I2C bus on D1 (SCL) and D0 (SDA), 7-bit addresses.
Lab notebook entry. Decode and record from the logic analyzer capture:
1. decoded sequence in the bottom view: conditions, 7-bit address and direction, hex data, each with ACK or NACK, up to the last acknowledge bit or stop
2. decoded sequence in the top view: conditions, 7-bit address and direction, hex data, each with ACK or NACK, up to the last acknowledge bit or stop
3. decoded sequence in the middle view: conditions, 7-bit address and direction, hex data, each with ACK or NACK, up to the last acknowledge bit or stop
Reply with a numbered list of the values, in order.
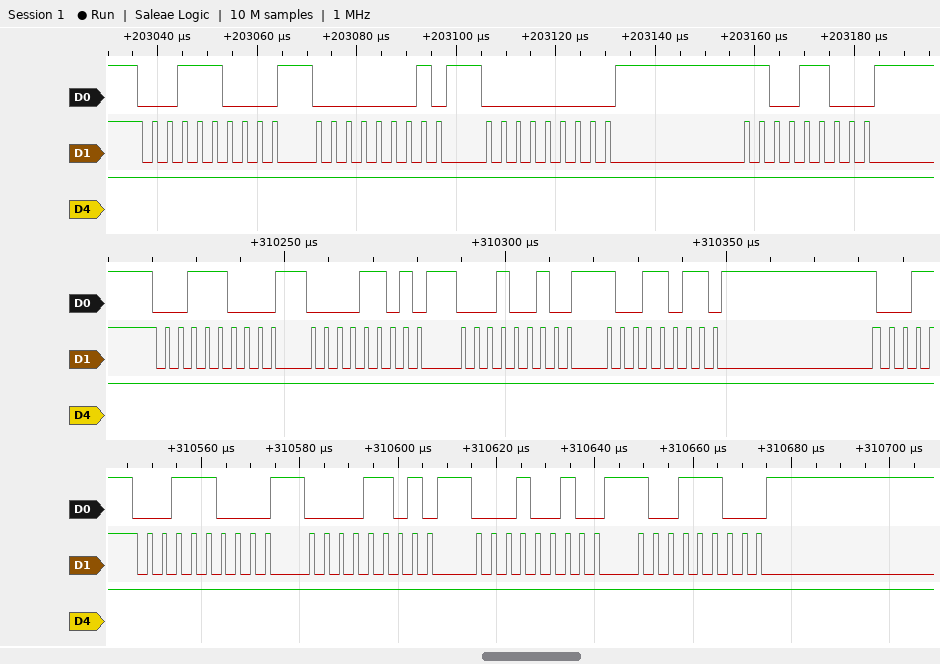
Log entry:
1. start, address 1C write ACK, 0D ACK, 12 ACK, 9C ACK
2. start, address 1C write ACK, 01 ACK, 00 ACK, CC ACK
3. start, address 1C write ACK, 0D ACK, 12 ACK, 9B ACK
